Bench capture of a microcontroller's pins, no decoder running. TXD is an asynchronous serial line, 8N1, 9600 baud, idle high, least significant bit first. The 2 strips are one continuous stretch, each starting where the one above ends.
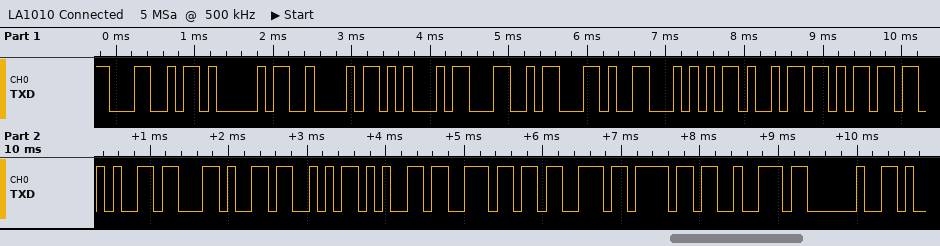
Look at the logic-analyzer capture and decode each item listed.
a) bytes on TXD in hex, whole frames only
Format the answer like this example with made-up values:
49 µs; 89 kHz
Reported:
0x4C 0x41 0x42 0x45 0x4C 0x2C 0x54 0x69 0x6D 0x65 0x2C 0x53 0x65 0x6E 0x73 0x6F 0x72 0x20
